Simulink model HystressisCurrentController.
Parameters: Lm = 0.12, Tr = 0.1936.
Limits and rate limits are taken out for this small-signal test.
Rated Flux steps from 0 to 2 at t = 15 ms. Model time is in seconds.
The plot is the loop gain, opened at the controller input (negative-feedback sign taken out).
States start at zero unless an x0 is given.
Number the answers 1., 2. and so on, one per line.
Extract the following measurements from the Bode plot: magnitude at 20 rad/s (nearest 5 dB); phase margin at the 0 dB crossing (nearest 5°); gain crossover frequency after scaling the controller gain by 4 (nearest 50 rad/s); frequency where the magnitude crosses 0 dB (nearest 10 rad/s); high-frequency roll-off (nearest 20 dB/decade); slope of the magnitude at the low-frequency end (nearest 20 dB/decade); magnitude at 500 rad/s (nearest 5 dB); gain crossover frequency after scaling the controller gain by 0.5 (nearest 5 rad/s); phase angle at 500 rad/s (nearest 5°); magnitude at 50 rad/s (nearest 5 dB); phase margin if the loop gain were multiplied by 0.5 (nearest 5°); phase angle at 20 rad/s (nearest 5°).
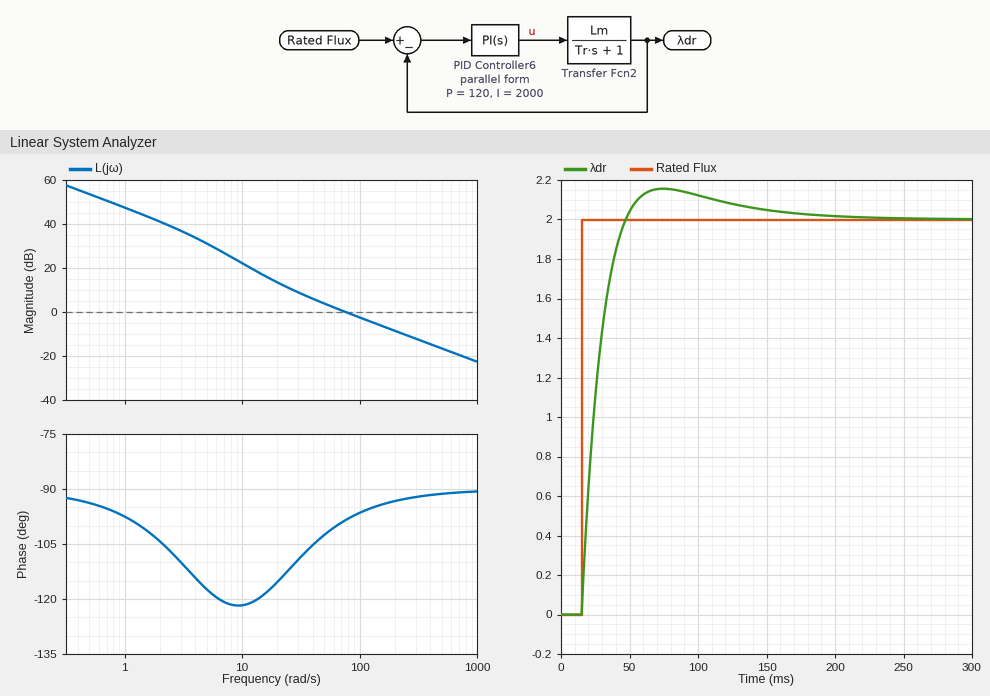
1. 15 dB
2. 80°
3. 300 rad/s
4. 80 rad/s
5. -20 dB/decade
6. -20 dB/decade
7. -15 dB
8. 40 rad/s
9. -90°
10. 5 dB
11. 75°
12. -115°
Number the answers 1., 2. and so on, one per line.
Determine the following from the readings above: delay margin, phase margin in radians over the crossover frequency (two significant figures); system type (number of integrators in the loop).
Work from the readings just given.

1. 0.017 s
2. 1
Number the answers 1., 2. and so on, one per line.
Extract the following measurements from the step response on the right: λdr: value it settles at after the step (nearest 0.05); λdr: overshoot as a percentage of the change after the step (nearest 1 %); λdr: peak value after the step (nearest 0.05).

1. 2.00
2. 8 %
3. 2.15
